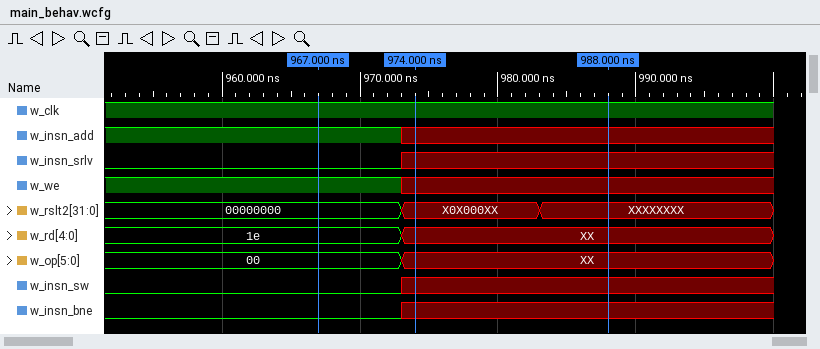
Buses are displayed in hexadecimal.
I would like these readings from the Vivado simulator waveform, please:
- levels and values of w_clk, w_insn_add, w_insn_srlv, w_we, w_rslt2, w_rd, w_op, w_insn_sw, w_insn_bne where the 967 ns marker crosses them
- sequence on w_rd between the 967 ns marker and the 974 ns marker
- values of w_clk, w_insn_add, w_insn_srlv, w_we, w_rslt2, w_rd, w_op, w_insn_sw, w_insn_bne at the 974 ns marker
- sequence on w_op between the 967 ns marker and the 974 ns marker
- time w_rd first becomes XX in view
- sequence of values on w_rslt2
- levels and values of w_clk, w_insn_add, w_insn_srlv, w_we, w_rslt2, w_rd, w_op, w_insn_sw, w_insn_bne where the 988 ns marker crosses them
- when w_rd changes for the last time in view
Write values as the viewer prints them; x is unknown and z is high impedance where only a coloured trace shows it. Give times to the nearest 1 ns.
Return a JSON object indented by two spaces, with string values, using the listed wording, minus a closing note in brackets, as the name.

{
  "levels and values of w_clk, w_insn_add, w_insn_srlv, w_we, w_rslt2, w_rd, w_op, w_insn_sw, w_insn_bne where the 967 ns marker crosses them": "w_clk=1, w_insn_add=1, w_insn_srlv=0, w_we=1, w_rslt2=00000000, w_rd=1e, w_op=00, w_insn_sw=0, w_insn_bne=0",
  "sequence on w_rd between the 967 ns marker and the 974 ns marker": "1e, XX",
  "values of w_clk, w_insn_add, w_insn_srlv, w_we, w_rslt2, w_rd, w_op, w_insn_sw, w_insn_bne at the 974 ns marker": "w_clk=1, w_insn_add=x, w_insn_srlv=x, w_we=x, w_rslt2=X0X000XX, w_rd=XX, w_op=XX, w_insn_sw=x, w_insn_bne=x",
  "sequence on w_op between the 967 ns marker and the 974 ns marker": "00, XX",
  "time w_rd first becomes XX in view": "973 ns",
  "sequence of values on w_rslt2": "00000000, X0X000XX, XXXXXXXX",
  "levels and values of w_clk, w_insn_add, w_insn_srlv, w_we, w_rslt2, w_rd, w_op, w_insn_sw, w_insn_bne where the 988 ns marker crosses them": "w_clk=1, w_insn_add=x, w_insn_srlv=x, w_we=x, w_rslt2=XXXXXXXX, w_rd=XX, w_op=XX, w_insn_sw=x, w_insn_bne=x",
  "when w_rd changes for the last time in view": "973 ns"
}
